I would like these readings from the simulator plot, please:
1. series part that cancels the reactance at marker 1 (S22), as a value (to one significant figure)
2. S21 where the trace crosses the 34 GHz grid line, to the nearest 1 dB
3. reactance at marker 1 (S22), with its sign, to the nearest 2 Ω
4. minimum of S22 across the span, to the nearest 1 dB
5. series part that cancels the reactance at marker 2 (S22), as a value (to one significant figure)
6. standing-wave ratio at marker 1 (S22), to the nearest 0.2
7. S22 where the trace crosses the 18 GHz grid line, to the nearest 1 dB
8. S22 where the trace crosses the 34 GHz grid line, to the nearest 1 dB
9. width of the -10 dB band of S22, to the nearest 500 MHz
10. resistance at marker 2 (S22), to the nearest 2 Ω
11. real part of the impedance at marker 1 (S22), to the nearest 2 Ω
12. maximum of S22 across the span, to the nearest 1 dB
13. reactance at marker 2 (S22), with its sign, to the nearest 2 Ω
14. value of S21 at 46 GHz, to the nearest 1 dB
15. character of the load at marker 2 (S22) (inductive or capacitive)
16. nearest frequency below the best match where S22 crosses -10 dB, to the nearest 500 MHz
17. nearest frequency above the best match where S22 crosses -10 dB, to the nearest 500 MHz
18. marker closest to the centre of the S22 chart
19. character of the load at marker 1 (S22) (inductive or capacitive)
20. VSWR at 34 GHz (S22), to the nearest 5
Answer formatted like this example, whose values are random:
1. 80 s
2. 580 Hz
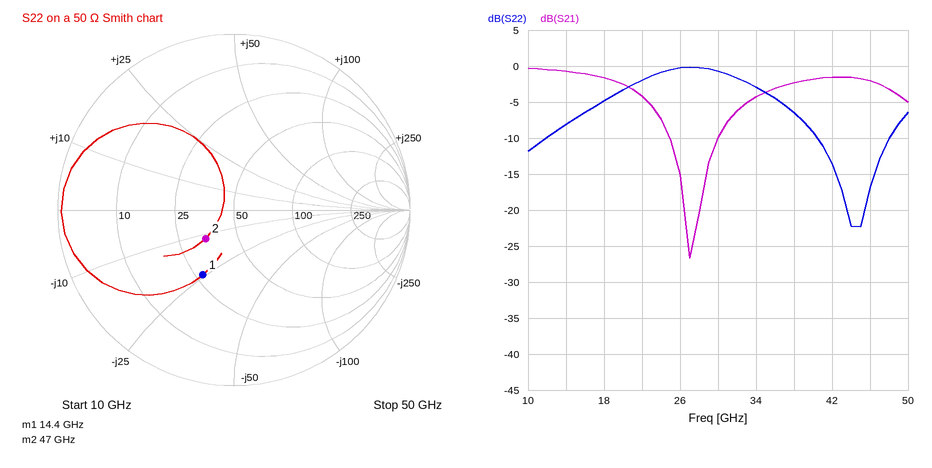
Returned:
1. 300 pH
2. -4 dB
3. -24 Ω
4. -22 dB
5. 40 pH
6. 2.4
7. -5 dB
8. -3 dB
9. 7.5 GHz
10. 34 Ω
11. 28 Ω
12. 0 dB
13. -12 Ω
14. -2 dB
15. capacitive
16. 40.5 GHz
17. 48.0 GHz
18. marker 2
19. capacitive
20. 5
